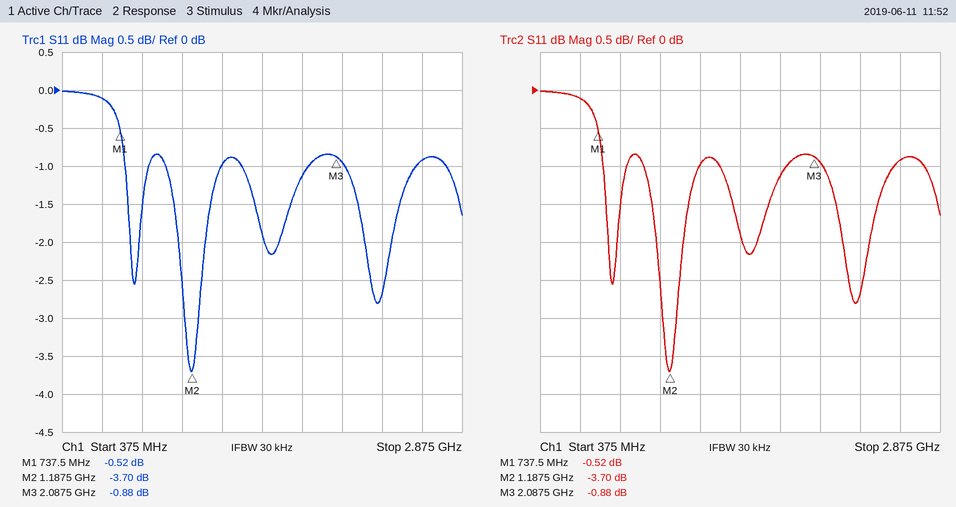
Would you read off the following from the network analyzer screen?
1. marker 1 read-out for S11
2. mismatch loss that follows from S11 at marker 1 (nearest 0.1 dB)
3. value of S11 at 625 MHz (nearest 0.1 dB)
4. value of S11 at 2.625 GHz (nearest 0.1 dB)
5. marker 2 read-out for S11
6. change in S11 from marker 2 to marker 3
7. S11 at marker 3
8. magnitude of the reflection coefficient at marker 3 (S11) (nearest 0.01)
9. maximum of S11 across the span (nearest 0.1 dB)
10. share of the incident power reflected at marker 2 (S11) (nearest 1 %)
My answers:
-0.52 dB
9.5 dB
-0.1 dB
-0.9 dB
-3.70 dB
2.82 dB
-0.88 dB
0.90
0.0 dB
43 %
